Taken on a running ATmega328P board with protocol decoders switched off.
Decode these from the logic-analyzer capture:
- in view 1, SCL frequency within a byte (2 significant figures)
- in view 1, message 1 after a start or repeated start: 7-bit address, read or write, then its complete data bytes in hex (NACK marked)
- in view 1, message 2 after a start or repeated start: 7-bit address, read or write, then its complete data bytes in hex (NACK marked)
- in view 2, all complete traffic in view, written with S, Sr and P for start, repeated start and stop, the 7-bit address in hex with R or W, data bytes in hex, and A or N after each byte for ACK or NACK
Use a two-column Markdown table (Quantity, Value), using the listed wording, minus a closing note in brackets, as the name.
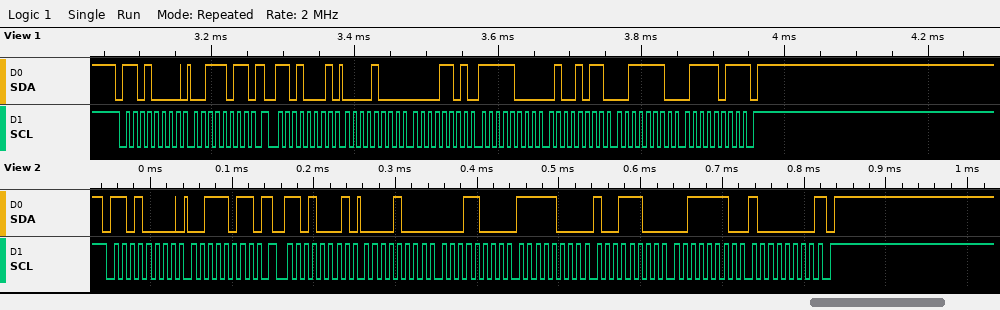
| Quantity | Value |
|---|---|
| in view 1, SCL frequency within a byte | 100 kHz |
| in view 1, message 1 after a start or repeated start: 7-bit address, read or write, then its complete data bytes in hex | 0x68 write: 3B |
| in view 1, message 2 after a start or repeated start: 7-bit address, read or write, then its complete data bytes in hex | 0x68 read: 08 0D F8 4B 3E 7B NACK |
| in view 2, all complete traffic in view, written with S, Sr and P for start, repeated start and stop, the 7-bit address in hex with R or W, data bytes in hex, and A or N after each byte for ACK or NACK | S 68W A 3B A Sr 68R A 08 A 18 A F8 A 9C A 3E A 80 N P |
